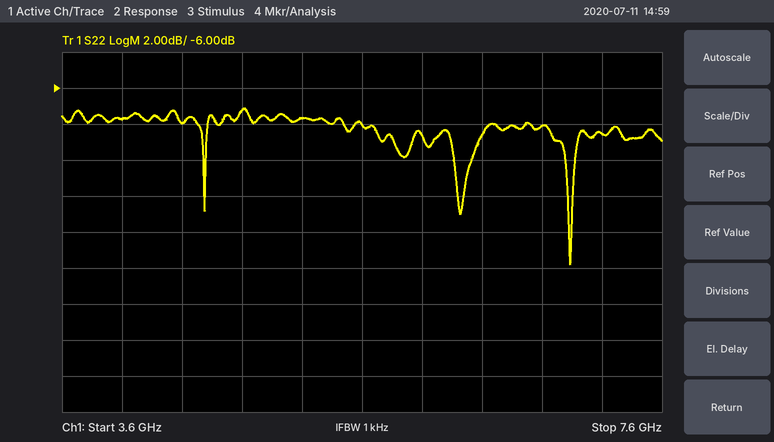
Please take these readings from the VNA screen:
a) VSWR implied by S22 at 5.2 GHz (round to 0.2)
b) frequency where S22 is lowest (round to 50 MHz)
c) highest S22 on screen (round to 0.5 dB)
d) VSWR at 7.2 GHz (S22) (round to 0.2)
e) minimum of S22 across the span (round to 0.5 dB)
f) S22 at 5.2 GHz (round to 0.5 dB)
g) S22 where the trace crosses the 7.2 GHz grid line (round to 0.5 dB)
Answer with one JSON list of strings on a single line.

["2.4", "7.00 GHz", "-7.0 dB", "2.2", "-16.0 dB", "-7.5 dB", "-8.5 dB"]
